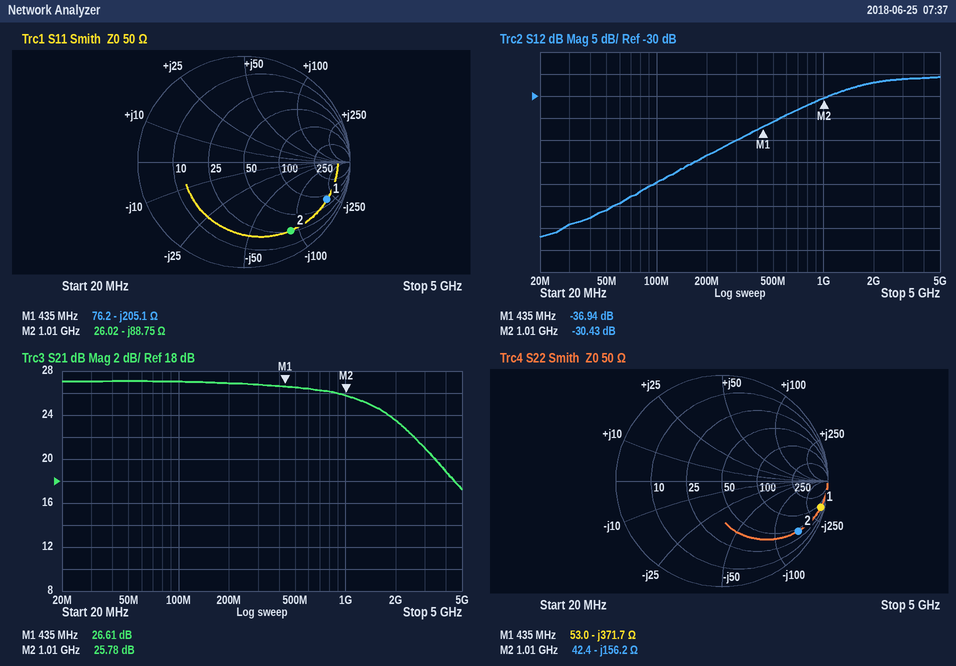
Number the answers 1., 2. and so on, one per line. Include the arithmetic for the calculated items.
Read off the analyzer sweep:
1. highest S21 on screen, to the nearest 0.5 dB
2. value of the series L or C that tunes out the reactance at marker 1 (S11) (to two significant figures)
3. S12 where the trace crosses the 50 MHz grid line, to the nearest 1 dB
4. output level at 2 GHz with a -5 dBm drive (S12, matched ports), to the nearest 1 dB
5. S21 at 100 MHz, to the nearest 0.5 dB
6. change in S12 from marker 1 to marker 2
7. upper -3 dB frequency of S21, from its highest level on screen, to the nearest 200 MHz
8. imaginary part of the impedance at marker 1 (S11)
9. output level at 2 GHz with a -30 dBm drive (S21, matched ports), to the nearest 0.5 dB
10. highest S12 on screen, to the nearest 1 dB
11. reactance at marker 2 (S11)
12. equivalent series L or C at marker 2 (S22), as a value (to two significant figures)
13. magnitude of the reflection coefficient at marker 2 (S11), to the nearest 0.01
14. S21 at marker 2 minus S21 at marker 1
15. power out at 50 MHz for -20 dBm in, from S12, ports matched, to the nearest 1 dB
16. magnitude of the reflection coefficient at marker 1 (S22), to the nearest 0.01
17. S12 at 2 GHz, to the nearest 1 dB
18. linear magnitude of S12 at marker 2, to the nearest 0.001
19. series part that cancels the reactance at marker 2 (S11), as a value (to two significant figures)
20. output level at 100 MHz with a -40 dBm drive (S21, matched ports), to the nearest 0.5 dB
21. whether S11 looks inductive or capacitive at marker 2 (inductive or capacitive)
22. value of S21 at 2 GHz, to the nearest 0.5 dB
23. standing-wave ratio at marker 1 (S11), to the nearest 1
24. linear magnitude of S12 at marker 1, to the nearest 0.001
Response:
1. 27.0 dB
2. L = 205.1 Ω/(2π × 435 MHz) ≈ 75 nH
3. -56 dB
4. -5 dBm + (-27 dB) = -32 dBm
5. 27.0 dB
6. -30.43 − (-36.94) = 6.51 dB
7. 1.8 GHz
8. -205.1 Ω
9. -30 dBm + (23.5 dB) = -6.5 dBm
10. -26 dB
11. -88.75 Ω
12. C = 1/(2π × 1.01 GHz × 156.2 Ω) ≈ 1.0 pF
13. 0.79
14. 25.78 − (26.61) = -0.83 dB
15. -20 dBm + (-56 dB) = -76 dBm
16. 0.96
17. -27 dB
18. 10^(-30.43/20) ≈ 0.030
19. L = 88.75 Ω/(2π × 1.01 GHz) ≈ 14 nH
20. -40 dBm + (27.0 dB) = -13.0 dBm
21. capacitive
22. 23.5 dB
23. 13
24. 10^(-36.94/20) ≈ 0.014
